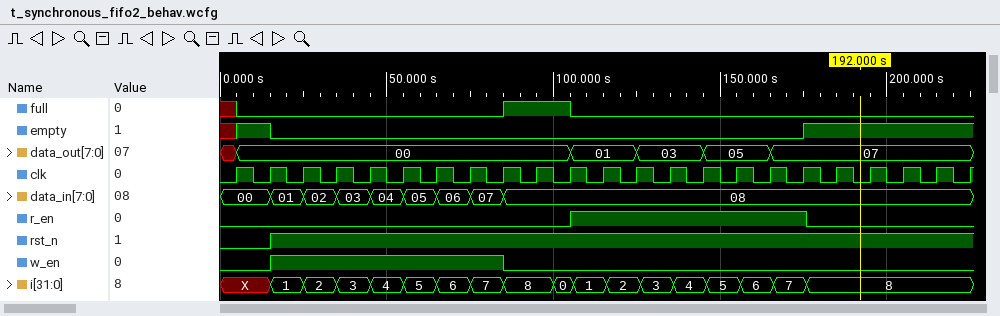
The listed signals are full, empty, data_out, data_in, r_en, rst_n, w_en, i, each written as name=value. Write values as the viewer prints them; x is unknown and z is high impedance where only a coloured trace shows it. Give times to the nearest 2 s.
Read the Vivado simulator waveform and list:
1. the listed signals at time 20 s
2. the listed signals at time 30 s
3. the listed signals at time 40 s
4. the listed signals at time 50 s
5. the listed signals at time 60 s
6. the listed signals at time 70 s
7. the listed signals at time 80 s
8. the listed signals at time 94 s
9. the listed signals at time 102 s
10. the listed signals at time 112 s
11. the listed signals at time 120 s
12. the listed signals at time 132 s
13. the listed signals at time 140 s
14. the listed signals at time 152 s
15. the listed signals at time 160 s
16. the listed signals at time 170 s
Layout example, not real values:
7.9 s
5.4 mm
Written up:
full=0, empty=0, data_out=00, data_in=01, r_en=0, rst_n=1, w_en=1, i=1
full=0, empty=0, data_out=00, data_in=02, r_en=0, rst_n=1, w_en=1, i=2
full=0, empty=0, data_out=00, data_in=03, r_en=0, rst_n=1, w_en=1, i=3
full=0, empty=0, data_out=00, data_in=04, r_en=0, rst_n=1, w_en=1, i=4
full=0, empty=0, data_out=00, data_in=05, r_en=0, rst_n=1, w_en=1, i=5
full=0, empty=0, data_out=00, data_in=06, r_en=0, rst_n=1, w_en=1, i=6
full=0, empty=0, data_out=00, data_in=07, r_en=0, rst_n=1, w_en=1, i=7
full=1, empty=0, data_out=00, data_in=08, r_en=0, rst_n=1, w_en=0, i=8
full=1, empty=0, data_out=00, data_in=08, r_en=0, rst_n=1, w_en=0, i=0
full=0, empty=0, data_out=01, data_in=08, r_en=1, rst_n=1, w_en=0, i=1
full=0, empty=0, data_out=01, data_in=08, r_en=1, rst_n=1, w_en=0, i=2
full=0, empty=0, data_out=03, data_in=08, r_en=1, rst_n=1, w_en=0, i=3
full=0, empty=0, data_out=03, data_in=08, r_en=1, rst_n=1, w_en=0, i=4
full=0, empty=0, data_out=05, data_in=08, r_en=1, rst_n=1, w_en=0, i=5
full=0, empty=0, data_out=05, data_in=08, r_en=1, rst_n=1, w_en=0, i=6
full=0, empty=0, data_out=07, data_in=08, r_en=1, rst_n=1, w_en=0, i=7
